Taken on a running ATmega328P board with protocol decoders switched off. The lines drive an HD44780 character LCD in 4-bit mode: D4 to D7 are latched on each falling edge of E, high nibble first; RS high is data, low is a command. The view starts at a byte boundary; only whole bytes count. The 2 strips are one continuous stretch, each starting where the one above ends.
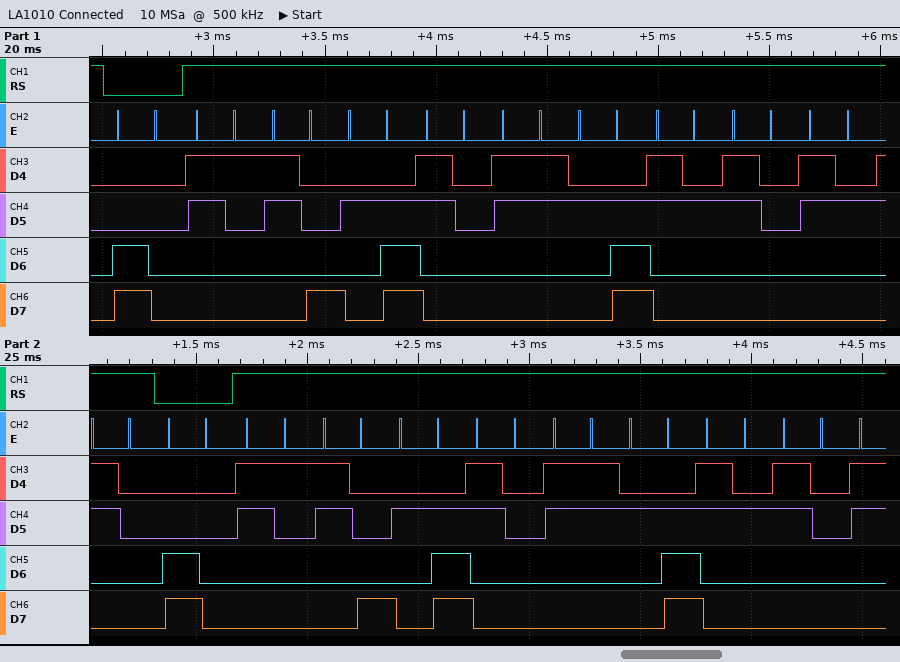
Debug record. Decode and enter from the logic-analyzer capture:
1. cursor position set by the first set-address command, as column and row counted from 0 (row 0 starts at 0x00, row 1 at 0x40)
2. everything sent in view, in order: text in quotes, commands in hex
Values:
column 0, row 1
0xC0 "18.03.2020" 0xC0 "18.03.20"
